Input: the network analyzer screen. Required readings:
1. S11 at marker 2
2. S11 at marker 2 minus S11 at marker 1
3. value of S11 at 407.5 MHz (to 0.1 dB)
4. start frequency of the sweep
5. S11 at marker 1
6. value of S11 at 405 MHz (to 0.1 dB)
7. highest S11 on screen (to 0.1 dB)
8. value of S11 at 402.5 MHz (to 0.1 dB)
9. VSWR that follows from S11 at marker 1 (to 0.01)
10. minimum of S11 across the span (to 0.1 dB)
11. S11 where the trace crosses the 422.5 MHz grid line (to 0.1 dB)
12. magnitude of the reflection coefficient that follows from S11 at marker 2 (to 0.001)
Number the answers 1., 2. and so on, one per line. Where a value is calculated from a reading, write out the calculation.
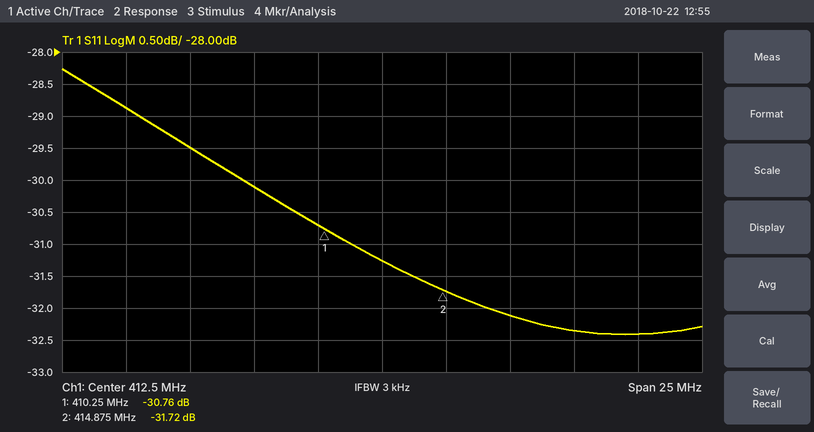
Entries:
1. -31.72 dB
2. -31.72 − (-30.76) = -0.96 dB
3. -30.1 dB
4. 400 MHz
5. -30.76 dB
6. -29.5 dB
7. -28.3 dB
8. -28.9 dB
9. (1 + 0.0290)/(1 − 0.0290) ≈ 1.06
10. -32.4 dB
11. -32.4 dB
12. 10^(-31.72/20) ≈ 0.026
